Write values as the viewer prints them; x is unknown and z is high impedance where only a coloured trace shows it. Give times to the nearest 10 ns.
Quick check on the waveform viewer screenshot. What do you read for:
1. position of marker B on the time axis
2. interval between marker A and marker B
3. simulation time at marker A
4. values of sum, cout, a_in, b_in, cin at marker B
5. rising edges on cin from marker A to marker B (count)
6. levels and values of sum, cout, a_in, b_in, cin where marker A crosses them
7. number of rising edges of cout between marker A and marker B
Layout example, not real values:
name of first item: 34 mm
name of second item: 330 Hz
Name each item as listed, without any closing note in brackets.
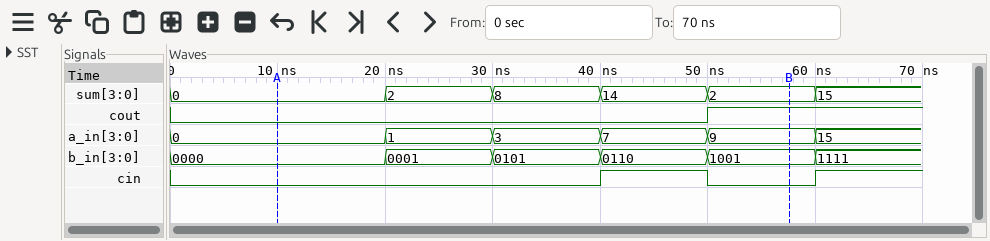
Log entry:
position of marker B on the time axis: 60 ns
interval between marker A and marker B: 50 ns
simulation time at marker A: 10 ns
values of sum, cout, a_in, b_in, cin at marker B: sum=2, cout=1, a_in=9, b_in=1001, cin=0
rising edges on cin from marker A to marker B: 1
levels and values of sum, cout, a_in, b_in, cin where marker A crosses them: sum=0, cout=0, a_in=0, b_in=0000, cin=0
number of rising edges of cout between marker A and marker B: 1
